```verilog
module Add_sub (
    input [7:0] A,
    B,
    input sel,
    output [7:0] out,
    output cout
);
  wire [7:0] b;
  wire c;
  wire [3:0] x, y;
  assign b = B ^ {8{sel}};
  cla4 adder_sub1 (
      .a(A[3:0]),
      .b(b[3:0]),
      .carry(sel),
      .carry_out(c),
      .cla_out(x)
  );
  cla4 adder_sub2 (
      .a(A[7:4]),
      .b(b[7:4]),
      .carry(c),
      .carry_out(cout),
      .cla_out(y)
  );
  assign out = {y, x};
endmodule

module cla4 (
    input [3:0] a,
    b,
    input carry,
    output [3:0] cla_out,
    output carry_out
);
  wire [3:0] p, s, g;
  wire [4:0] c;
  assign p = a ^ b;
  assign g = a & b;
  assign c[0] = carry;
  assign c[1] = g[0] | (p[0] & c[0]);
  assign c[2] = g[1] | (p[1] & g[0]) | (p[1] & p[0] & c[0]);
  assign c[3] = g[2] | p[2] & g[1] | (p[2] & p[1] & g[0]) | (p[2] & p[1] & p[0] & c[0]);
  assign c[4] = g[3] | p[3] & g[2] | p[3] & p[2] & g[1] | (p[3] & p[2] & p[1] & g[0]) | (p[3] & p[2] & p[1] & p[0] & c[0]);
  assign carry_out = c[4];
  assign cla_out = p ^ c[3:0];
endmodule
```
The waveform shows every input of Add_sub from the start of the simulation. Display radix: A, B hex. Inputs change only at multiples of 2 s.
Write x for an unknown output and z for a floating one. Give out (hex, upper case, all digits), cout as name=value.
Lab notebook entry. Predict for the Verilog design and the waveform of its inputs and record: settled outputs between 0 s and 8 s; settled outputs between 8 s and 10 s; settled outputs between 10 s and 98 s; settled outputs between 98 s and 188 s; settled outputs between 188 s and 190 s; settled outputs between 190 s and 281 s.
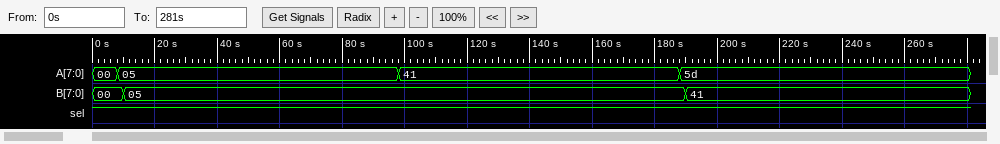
out=00, cout=1
out=05, cout=1
out=00, cout=1
out=3C, cout=1
out=58, cout=1
out=1C, cout=1
